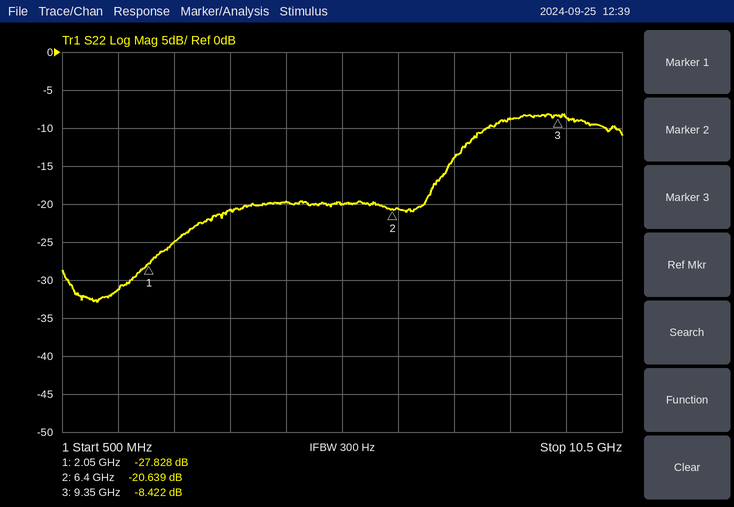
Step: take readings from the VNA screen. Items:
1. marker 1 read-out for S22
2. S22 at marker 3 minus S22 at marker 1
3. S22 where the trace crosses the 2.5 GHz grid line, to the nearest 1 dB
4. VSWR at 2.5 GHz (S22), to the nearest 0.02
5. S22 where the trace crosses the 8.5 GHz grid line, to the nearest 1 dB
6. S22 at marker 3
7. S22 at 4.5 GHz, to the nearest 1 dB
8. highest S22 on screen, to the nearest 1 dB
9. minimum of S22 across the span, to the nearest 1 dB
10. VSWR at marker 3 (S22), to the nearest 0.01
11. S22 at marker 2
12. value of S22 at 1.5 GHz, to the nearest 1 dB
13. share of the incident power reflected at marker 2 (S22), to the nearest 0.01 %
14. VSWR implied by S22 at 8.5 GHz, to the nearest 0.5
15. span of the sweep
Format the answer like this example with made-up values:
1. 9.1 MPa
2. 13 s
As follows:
1. -27.828 dB
2. 19.406 dB
3. -25 dB
4. 1.12
5. -9 dB
6. -8.422 dB
7. -20 dB
8. -8 dB
9. -33 dB
10. 2.22
11. -20.639 dB
12. -31 dB
13. 0.86 %
14. 2.0
15. 10 GHz
